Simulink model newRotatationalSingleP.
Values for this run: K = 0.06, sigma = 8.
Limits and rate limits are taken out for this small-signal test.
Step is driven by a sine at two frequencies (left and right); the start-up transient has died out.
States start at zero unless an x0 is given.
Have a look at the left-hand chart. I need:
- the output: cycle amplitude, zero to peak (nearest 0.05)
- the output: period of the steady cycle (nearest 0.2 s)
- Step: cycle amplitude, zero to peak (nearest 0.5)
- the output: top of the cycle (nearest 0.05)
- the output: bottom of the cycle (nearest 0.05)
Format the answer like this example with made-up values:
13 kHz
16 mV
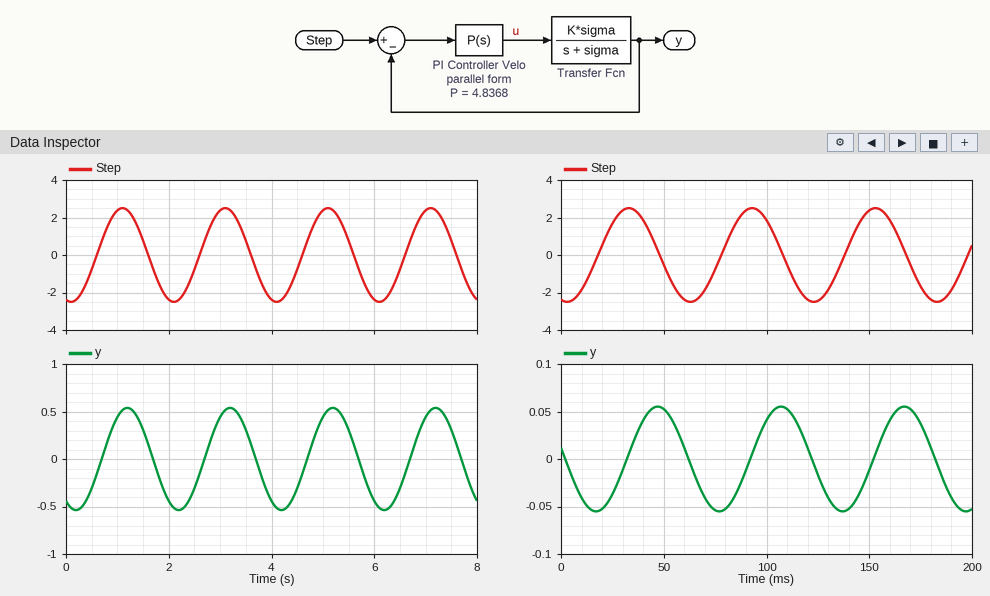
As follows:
0.55
2.0 s
2.5
0.55
-0.55
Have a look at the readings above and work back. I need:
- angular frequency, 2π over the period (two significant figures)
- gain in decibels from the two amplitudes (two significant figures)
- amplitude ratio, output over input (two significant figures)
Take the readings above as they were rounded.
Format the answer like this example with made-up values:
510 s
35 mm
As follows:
3.1 rad/s
-13 dB
0.22
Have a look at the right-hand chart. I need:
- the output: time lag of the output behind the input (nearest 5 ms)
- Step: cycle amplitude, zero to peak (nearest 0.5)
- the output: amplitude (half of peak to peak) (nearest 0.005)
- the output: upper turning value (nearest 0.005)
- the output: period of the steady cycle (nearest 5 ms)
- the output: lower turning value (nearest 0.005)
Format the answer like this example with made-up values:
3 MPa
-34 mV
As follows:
15 ms
2.5
0.055
0.055
60 ms
-0.055
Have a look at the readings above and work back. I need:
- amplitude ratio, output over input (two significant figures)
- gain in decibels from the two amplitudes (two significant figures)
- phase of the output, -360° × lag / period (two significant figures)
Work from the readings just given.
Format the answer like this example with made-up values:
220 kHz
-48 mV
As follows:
0.022
-33 dB
-90°
